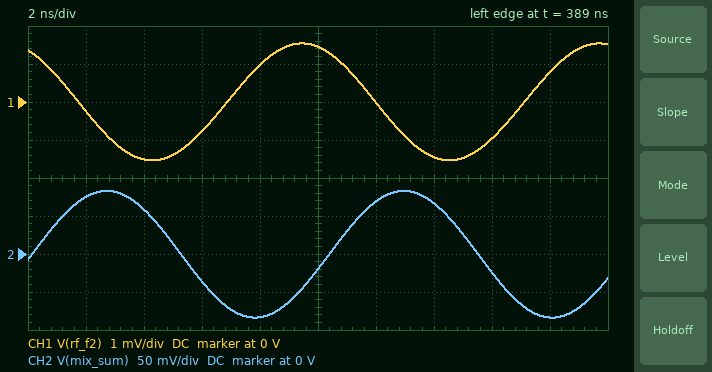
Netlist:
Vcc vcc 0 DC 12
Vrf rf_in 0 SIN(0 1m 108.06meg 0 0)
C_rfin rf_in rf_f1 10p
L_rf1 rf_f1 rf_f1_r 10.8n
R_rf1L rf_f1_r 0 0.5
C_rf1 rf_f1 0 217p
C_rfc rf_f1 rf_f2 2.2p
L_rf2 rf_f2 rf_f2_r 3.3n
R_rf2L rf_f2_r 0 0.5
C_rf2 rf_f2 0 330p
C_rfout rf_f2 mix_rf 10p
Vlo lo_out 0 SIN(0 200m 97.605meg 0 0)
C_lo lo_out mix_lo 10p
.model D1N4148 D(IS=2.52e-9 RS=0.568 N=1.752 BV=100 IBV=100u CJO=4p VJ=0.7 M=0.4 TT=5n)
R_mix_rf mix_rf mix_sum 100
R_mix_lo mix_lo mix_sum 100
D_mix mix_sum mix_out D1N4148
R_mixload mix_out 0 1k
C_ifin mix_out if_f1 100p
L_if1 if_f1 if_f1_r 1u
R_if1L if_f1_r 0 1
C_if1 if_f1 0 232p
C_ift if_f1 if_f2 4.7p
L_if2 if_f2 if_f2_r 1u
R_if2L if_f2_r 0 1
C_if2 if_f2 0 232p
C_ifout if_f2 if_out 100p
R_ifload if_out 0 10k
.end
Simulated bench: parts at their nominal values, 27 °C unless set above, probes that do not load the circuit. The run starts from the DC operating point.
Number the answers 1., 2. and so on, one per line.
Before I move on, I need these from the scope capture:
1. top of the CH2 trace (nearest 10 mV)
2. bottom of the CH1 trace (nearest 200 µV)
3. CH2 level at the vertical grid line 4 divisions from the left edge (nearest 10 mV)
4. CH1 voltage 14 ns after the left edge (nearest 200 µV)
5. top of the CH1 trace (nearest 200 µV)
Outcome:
1. 80 mV
2. -1.6 mV
3. -80 mV
4. -1.4 mV
5. 1.6 mV
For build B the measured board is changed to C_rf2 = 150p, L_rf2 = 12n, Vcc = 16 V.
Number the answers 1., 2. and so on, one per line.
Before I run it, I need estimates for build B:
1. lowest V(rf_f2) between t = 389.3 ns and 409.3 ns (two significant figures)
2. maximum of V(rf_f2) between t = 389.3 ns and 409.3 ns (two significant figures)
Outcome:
1. -11 mV
2. 11 mV
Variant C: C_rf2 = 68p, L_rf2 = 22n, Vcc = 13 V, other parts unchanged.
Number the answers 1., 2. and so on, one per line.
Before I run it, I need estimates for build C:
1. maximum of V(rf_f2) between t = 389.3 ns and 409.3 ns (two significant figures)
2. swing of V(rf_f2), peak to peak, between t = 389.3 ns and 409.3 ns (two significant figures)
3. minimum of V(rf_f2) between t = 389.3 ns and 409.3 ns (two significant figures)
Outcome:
1. 15 mV
2. 31 mV
3. -15 mV
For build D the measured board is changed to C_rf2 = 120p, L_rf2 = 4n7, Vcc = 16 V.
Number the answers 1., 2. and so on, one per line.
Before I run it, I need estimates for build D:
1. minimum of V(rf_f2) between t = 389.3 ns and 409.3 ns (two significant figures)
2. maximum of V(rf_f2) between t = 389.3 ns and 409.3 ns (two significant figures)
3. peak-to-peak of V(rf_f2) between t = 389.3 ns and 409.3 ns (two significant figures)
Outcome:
1. -1.6 mV
2. 1.7 mV
3. 3.3 mV
